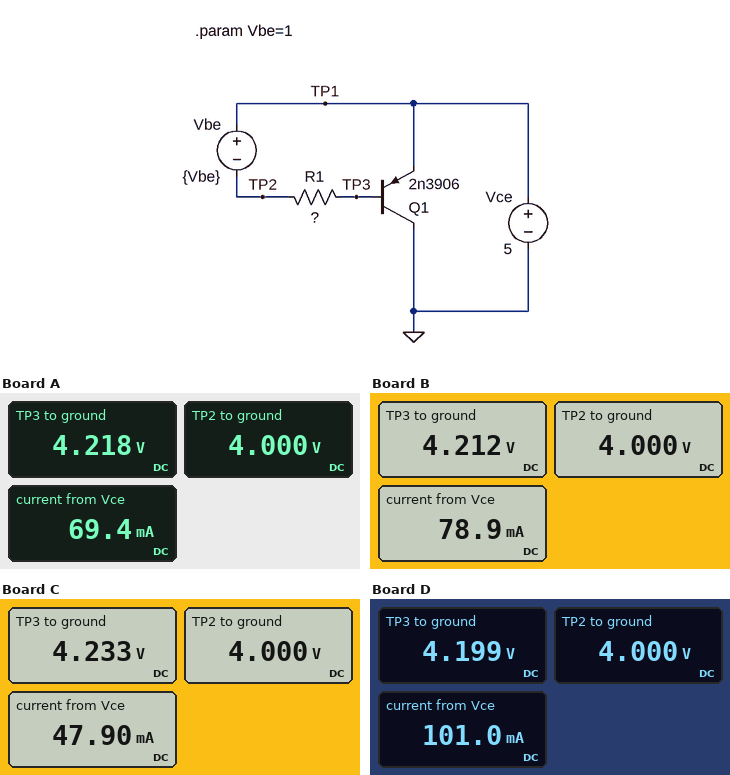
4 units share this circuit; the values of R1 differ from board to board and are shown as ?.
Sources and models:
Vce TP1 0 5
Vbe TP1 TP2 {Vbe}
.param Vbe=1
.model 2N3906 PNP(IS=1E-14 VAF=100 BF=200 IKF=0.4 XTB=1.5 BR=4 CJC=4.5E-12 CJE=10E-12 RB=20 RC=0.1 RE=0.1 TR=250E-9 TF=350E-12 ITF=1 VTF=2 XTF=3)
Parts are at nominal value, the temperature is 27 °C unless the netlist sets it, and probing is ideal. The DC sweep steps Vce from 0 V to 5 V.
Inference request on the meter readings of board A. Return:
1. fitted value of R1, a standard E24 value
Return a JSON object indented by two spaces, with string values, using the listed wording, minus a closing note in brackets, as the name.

{
  "fitted value of R1, a standard E24 value": "560 Ω"
}
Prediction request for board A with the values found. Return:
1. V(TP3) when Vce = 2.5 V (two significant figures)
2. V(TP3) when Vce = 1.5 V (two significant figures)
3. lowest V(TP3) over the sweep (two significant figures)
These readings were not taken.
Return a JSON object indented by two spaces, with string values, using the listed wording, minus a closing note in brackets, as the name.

{
  "V(TP3) when Vce = 2.5 V": "1.7 V",
  "V(TP3) when Vce = 1.5 V": "720 mV",
  "lowest V(TP3) over the sweep": "-690 mV"
}
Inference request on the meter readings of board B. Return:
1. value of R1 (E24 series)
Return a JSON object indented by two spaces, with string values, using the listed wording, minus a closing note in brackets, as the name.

{
  "value of R1": "470 Ω"
}
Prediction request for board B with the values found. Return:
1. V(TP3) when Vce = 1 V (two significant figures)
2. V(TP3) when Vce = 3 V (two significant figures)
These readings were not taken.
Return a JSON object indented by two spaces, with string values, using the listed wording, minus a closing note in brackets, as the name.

{
  "V(TP3) when Vce = 1 V": "210 mV",
  "V(TP3) when Vce = 3 V": "2.2 V"
}
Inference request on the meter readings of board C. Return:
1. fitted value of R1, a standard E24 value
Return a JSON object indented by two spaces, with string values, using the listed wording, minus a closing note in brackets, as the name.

{
  "fitted value of R1, a standard E24 value": "910 Ω"
}
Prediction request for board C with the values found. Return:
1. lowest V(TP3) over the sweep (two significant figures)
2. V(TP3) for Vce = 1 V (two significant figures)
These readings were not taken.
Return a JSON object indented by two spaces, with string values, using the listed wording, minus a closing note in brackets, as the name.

{
  "lowest V(TP3) over the sweep": "-670 mV",
  "V(TP3) for Vce = 1 V": "230 mV"
}
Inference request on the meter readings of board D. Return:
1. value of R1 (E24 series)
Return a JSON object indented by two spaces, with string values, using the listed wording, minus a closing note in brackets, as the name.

{
  "value of R1": "330 Ω"
}
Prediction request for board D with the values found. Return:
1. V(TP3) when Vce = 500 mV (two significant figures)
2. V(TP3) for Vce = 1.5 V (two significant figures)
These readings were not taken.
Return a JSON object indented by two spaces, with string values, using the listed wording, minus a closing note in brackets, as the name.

{
  "V(TP3) when Vce = 500 mV": "-300 mV",
  "V(TP3) for Vce = 1.5 V": "700 mV"
}
